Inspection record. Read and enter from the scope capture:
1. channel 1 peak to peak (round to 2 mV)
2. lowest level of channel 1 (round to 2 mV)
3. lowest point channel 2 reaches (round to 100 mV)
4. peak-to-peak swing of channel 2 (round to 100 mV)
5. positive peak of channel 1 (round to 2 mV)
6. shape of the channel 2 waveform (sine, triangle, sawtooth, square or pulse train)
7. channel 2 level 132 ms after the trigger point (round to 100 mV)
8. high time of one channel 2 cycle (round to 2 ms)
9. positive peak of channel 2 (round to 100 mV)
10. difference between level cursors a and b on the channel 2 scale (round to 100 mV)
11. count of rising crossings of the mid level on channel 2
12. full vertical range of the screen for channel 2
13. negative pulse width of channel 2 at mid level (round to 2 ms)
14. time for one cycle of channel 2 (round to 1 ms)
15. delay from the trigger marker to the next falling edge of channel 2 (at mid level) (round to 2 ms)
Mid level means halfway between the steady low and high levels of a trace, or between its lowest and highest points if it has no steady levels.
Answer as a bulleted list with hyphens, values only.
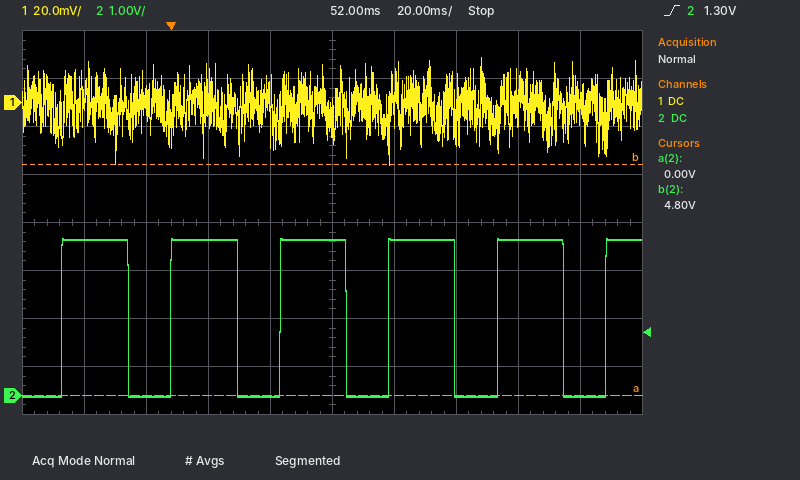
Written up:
- 44 mV
- -26 mV
- 0.0 V
- 3.3 V
- 18 mV
- pulse train
- 0.0 V
- 22 ms
- 3.3 V
- 4.8 V
- 6
- 8 V
- 14 ms
- 35 ms
- 22 ms
